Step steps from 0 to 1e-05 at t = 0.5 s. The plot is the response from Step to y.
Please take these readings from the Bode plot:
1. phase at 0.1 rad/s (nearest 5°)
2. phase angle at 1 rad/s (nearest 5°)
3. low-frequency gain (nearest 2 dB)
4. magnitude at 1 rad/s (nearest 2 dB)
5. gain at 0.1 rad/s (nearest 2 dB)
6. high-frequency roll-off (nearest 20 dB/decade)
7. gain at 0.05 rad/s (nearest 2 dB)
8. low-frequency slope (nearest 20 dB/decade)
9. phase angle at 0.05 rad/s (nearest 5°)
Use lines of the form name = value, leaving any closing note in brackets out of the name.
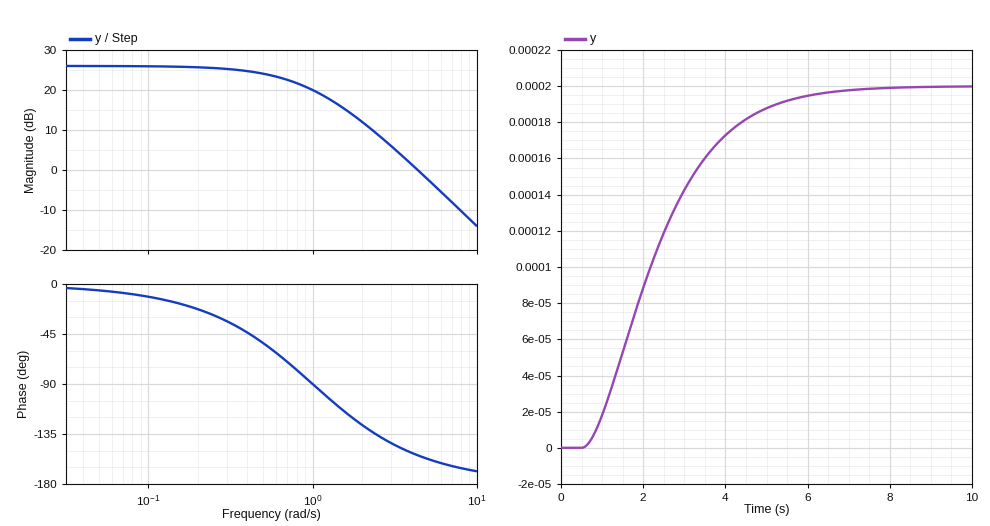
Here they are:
phase at 0.1 rad/s = -10°
phase angle at 1 rad/s = -90°
low-frequency gain = 26 dB
magnitude at 1 rad/s = 20 dB
gain at 0.1 rad/s = 26 dB
high-frequency roll-off = -40 dB/decade
gain at 0.05 rad/s = 26 dB
low-frequency slope = 0 dB/decade
phase angle at 0.05 rad/s = -5°
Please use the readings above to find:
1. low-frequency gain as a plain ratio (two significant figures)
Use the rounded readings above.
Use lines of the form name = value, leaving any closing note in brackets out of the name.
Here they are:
low-frequency gain as a plain ratio = 20
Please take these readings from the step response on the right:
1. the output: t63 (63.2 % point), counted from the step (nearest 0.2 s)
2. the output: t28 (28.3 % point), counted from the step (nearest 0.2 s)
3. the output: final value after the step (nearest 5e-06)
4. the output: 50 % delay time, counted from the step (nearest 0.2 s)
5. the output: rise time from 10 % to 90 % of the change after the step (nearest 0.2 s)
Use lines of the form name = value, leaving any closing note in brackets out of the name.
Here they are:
the output: t63 (63.2 % point), counted from the step = 2.2 s
the output: t28 (28.3 % point), counted from the step = 1.0 s
the output: final value after the step = 0.000200
the output: 50 % delay time, counted from the step = 1.6 s
the output: rise time from 10 % to 90 % of the change after the step = 3.4 s
